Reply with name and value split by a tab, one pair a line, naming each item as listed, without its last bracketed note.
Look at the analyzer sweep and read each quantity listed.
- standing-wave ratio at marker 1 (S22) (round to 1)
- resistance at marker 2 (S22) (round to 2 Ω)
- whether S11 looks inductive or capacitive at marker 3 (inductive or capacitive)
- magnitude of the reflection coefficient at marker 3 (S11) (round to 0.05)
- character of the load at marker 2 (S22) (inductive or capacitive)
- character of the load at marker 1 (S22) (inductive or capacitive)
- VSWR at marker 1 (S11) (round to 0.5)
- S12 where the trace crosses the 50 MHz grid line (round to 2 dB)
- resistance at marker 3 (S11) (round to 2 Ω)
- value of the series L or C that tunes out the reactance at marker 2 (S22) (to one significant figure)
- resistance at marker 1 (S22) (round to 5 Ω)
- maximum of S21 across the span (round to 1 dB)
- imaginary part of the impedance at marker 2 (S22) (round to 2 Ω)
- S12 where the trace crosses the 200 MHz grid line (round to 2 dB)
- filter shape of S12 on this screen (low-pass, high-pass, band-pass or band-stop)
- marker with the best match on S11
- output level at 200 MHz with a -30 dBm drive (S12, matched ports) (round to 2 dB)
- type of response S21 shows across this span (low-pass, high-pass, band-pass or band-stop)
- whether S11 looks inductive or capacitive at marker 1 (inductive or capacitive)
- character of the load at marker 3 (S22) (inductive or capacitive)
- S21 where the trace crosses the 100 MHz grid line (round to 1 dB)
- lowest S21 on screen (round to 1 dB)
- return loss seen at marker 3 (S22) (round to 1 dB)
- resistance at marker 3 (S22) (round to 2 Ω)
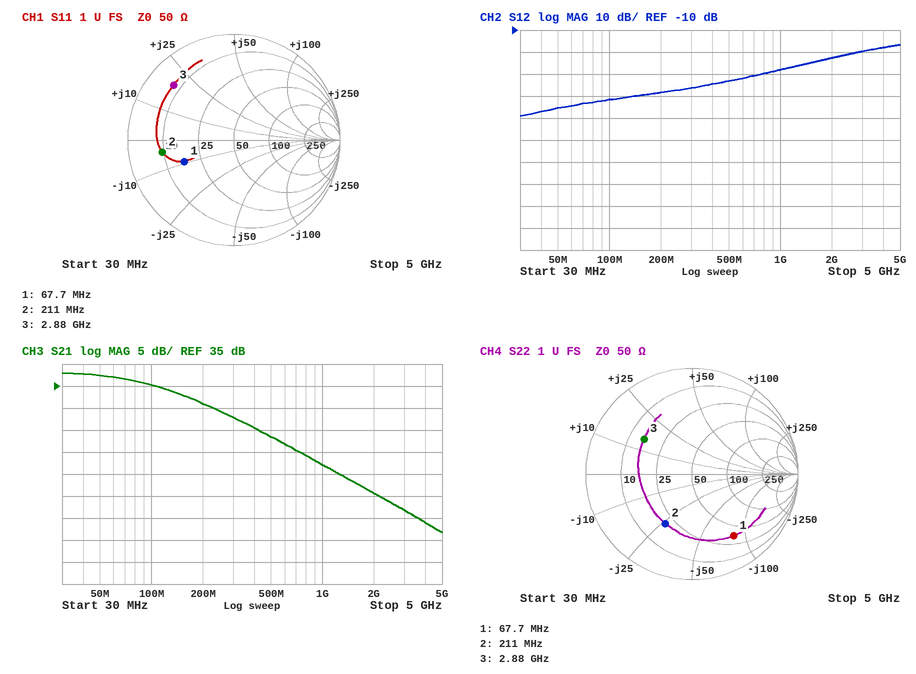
standing-wave ratio at marker 1 (S22)	6
resistance at marker 2 (S22)	20 Ω
whether S11 looks inductive or capacitive at marker 3	inductive
magnitude of the reflection coefficient at marker 3 (S11)	0.75
character of the load at marker 2 (S22)	capacitive
character of the load at marker 1 (S22)	capacitive
VSWR at marker 1 (S11)	3.0
S12 where the trace crosses the 50 MHz grid line	-46 dB
resistance at marker 3 (S11)	8 Ω
value of the series L or C that tunes out the reactance at marker 2 (S22)	20 nH
resistance at marker 1 (S22)	35 Ω
maximum of S21 across the span	38 dB
imaginary part of the impedance at marker 2 (S22)	-26 Ω
S12 where the trace crosses the 200 MHz grid line	-38 dB
filter shape of S12 on this screen	high-pass
marker with the best match on S11	marker 1
output level at 200 MHz with a -30 dBm drive (S12, matched ports)	-68 dBm
type of response S21 shows across this span	low-pass
whether S11 looks inductive or capacitive at marker 1	capacitive
character of the load at marker 3 (S22)	inductive
S21 where the trace crosses the 100 MHz grid line	35 dB
lowest S21 on screen	2 dB
return loss seen at marker 3 (S22)	5 dB
resistance at marker 3 (S22)	16 Ω
